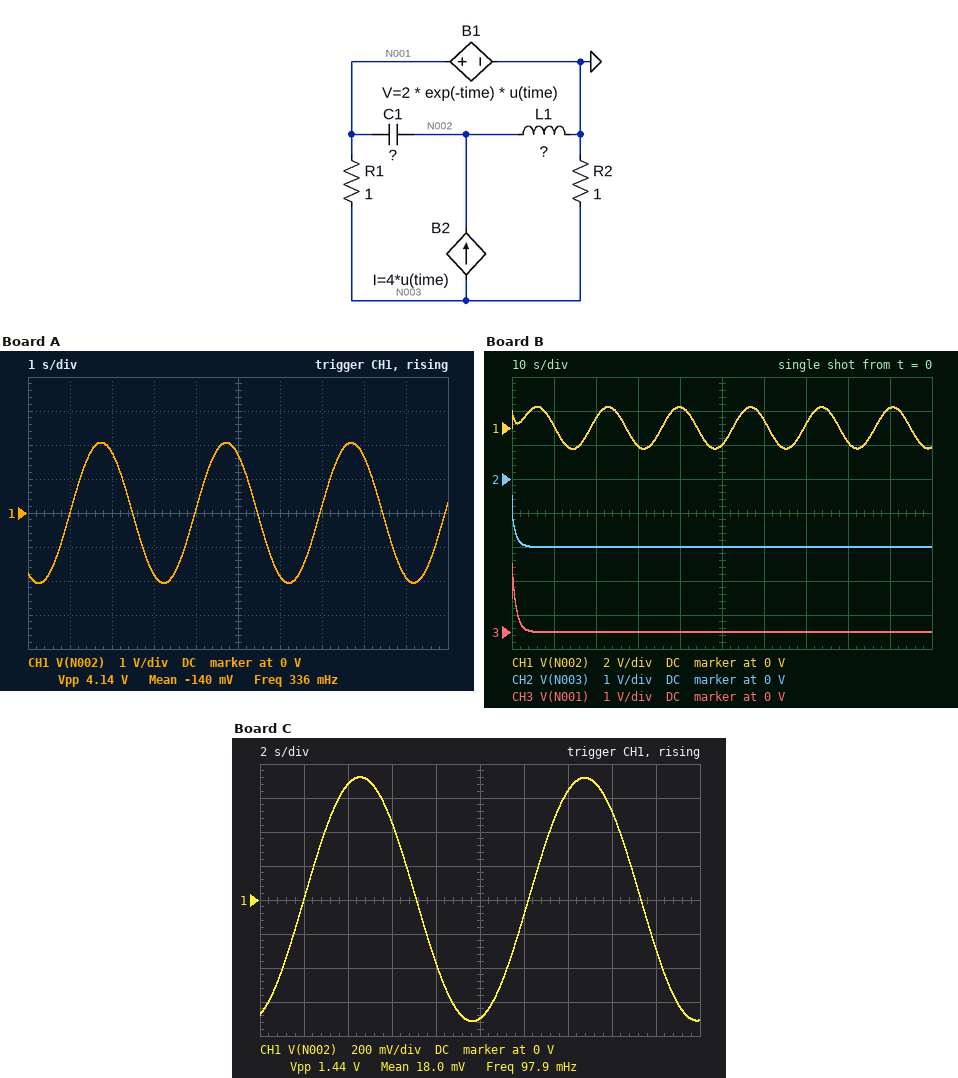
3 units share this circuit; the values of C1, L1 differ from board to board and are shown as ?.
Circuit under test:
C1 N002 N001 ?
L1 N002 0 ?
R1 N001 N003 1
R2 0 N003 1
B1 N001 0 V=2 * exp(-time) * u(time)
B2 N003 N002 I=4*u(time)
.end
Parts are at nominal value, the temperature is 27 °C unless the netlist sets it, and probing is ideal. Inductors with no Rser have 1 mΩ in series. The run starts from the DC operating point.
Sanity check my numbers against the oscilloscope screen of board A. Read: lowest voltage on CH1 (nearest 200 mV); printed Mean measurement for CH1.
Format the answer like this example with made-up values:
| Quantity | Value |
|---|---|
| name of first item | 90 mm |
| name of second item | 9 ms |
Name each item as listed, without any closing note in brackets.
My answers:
| Quantity | Value |
|---|---|
| lowest voltage on CH1 | -2.0 V |
| printed Mean measurement for CH1 | -140 mV |
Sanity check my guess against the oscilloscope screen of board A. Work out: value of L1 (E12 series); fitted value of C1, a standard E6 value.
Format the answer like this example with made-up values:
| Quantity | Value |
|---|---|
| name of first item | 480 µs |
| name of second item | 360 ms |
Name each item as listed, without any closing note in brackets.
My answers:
| Quantity | Value |
|---|---|
| value of L1 | 680 mH |
| fitted value of C1, a standard E6 value | 330 mF |
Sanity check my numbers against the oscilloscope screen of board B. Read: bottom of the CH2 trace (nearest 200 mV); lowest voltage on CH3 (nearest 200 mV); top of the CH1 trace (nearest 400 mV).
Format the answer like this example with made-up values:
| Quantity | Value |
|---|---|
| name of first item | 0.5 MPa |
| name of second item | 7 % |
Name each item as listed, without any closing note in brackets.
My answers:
| Quantity | Value |
|---|---|
| bottom of the CH2 trace | -2.0 V |
| lowest voltage on CH3 | 0 V |
| top of the CH1 trace | 1.2 V |
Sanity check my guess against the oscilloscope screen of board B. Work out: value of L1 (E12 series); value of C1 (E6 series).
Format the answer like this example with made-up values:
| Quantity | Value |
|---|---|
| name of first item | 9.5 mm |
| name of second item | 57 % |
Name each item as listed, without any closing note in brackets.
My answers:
| Quantity | Value |
|---|---|
| value of L1 | 2.2 H |
| value of C1 | 3.3 F |
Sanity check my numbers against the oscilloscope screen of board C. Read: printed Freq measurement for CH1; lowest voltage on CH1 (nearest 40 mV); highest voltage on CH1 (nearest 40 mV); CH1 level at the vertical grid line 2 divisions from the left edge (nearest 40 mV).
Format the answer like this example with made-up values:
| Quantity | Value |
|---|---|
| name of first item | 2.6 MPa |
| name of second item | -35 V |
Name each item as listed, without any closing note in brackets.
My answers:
| Quantity | Value |
|---|---|
| printed Freq measurement for CH1 | 97.9 mHz |
| lowest voltage on CH1 | -720 mV |
| highest voltage on CH1 | 720 mV |
| CH1 level at the vertical grid line 2 divisions from the left edge | 680 mV |
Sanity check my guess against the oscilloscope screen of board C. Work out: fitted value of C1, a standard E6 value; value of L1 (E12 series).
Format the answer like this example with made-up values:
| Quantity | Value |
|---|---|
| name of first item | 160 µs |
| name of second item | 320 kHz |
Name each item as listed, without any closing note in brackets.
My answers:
| Quantity | Value |
|---|---|
| fitted value of C1, a standard E6 value | 2.2 F |
| value of L1 | 1.2 H |
